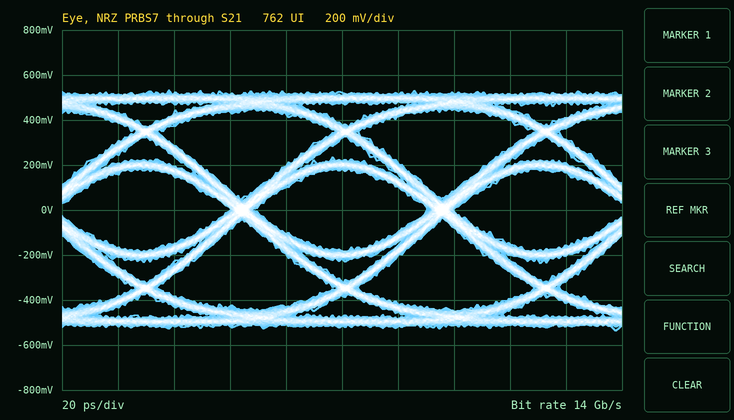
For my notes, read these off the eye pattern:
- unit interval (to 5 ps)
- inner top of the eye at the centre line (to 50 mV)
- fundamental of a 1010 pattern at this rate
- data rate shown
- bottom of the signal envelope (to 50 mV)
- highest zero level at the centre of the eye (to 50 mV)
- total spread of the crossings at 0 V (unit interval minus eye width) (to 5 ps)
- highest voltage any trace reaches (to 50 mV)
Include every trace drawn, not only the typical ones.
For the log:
70 ps
200 mV
7 GHz
14 Gb/s
-550 mV
-200 mV
10 ps
550 mV
